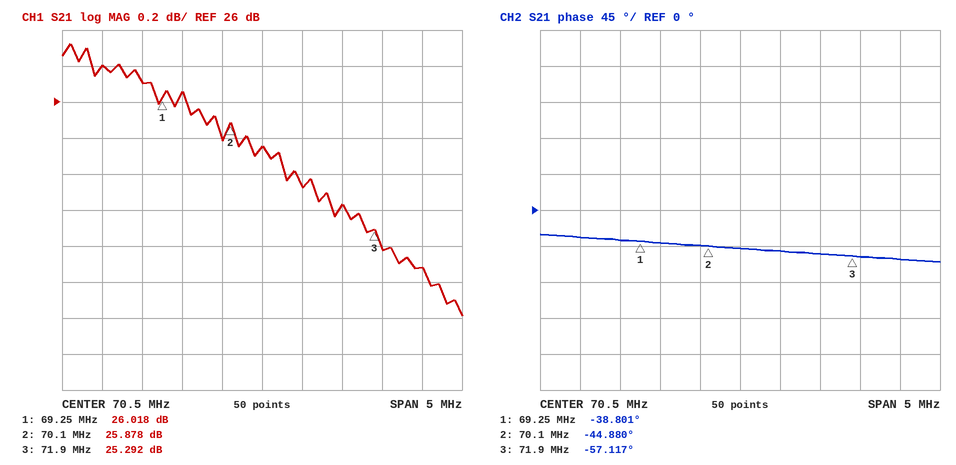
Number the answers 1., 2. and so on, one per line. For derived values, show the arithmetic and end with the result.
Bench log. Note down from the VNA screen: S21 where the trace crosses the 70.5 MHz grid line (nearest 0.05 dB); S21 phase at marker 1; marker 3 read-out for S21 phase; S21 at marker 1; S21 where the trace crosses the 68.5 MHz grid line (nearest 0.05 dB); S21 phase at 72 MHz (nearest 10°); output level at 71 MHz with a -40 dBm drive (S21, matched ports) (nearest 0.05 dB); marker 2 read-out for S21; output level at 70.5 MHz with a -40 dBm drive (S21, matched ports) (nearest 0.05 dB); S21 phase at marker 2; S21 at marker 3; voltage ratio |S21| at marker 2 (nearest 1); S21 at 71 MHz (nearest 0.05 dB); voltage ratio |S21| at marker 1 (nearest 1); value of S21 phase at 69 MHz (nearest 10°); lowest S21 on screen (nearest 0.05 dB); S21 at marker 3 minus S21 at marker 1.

1. 25.75 dB
2. -38.801°
3. -57.117°
4. 26.018 dB
5. 26.20 dB
6. -60°
7. -40 dBm + (25.55 dB) = -14.45 dBm
8. 25.878 dB
9. -40 dBm + (25.75 dB) = -14.25 dBm
10. -44.880°
11. 25.292 dB
12. 10^(25.878/20) ≈ 20
13. 25.55 dB
14. 10^(26.018/20) ≈ 20
15. -40°
16. 24.80 dB
17. 25.292 − (26.018) = -0.726 dB
